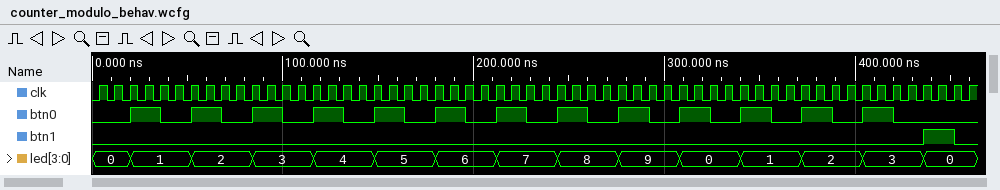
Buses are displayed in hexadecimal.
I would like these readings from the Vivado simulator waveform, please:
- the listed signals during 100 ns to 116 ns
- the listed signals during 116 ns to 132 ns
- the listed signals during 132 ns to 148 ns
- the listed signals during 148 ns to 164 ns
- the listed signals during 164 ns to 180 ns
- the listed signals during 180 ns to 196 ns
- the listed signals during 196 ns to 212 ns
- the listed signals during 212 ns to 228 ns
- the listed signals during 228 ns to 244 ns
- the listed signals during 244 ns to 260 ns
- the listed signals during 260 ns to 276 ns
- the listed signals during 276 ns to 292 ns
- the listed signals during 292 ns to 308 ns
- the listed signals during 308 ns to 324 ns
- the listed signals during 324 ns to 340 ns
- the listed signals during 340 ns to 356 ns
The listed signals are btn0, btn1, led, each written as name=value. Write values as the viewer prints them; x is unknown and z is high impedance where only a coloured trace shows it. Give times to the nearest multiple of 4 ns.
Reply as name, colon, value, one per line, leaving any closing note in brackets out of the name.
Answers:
the listed signals during 100 ns to 116 ns: btn0=0, btn1=0, led=3
the listed signals during 116 ns to 132 ns: btn0=1, btn1=0, led=4
the listed signals during 132 ns to 148 ns: btn0=0, btn1=0, led=4
the listed signals during 148 ns to 164 ns: btn0=1, btn1=0, led=5
the listed signals during 164 ns to 180 ns: btn0=0, btn1=0, led=5
the listed signals during 180 ns to 196 ns: btn0=1, btn1=0, led=6
the listed signals during 196 ns to 212 ns: btn0=0, btn1=0, led=6
the listed signals during 212 ns to 228 ns: btn0=1, btn1=0, led=7
the listed signals during 228 ns to 244 ns: btn0=0, btn1=0, led=7
the listed signals during 244 ns to 260 ns: btn0=1, btn1=0, led=8
the listed signals during 260 ns to 276 ns: btn0=0, btn1=0, led=8
the listed signals during 276 ns to 292 ns: btn0=1, btn1=0, led=9
the listed signals during 292 ns to 308 ns: btn0=0, btn1=0, led=9
the listed signals during 308 ns to 324 ns: btn0=1, btn1=0, led=0
the listed signals during 324 ns to 340 ns: btn0=0, btn1=0, led=0
the listed signals during 340 ns to 356 ns: btn0=1, btn1=0, led=1
